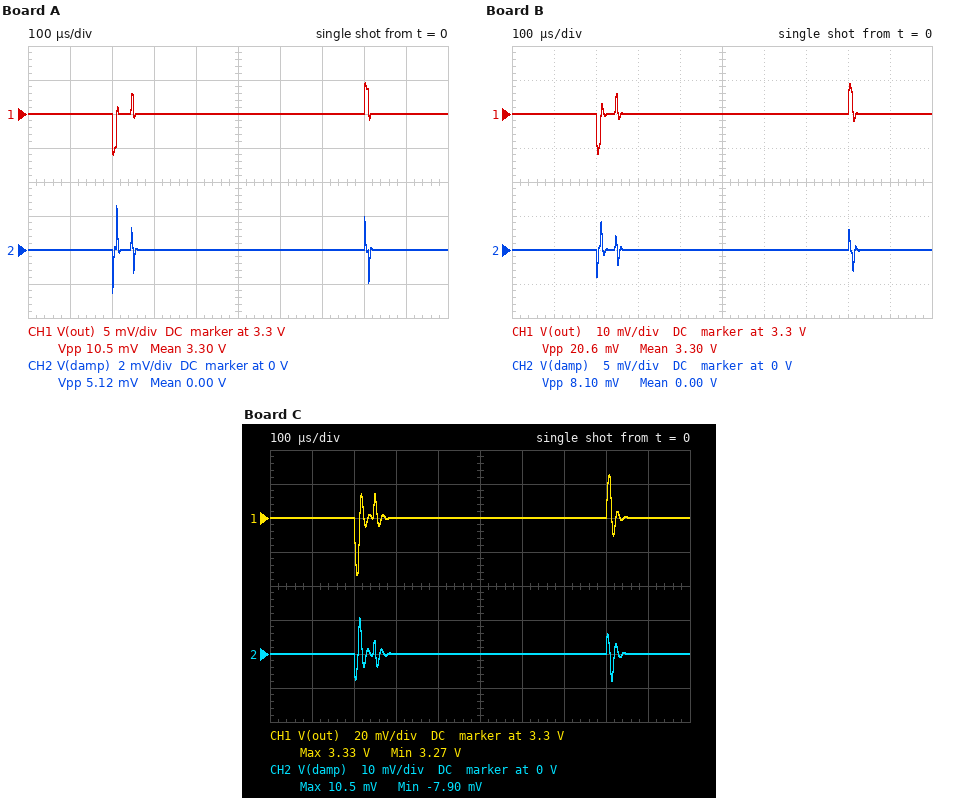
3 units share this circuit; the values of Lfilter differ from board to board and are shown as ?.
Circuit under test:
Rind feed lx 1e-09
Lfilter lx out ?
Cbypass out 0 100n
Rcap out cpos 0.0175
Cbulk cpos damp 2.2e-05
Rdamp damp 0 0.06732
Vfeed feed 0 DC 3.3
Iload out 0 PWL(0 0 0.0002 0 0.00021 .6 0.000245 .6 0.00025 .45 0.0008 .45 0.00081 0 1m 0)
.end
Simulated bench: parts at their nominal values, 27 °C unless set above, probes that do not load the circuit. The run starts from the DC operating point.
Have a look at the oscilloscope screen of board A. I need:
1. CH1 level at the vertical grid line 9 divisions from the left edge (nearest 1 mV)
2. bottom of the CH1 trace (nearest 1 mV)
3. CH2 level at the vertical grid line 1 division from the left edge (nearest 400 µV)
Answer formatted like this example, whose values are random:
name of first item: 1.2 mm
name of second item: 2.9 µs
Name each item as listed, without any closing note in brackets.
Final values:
CH1 level at the vertical grid line 9 divisions from the left edge: 3.300 V
bottom of the CH1 trace: 3.294 V
CH2 level at the vertical grid line 1 division from the left edge: 0 V
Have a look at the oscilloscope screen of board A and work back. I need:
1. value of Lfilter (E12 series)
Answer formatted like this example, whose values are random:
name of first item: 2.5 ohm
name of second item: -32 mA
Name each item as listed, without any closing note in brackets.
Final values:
value of Lfilter: 82 nH
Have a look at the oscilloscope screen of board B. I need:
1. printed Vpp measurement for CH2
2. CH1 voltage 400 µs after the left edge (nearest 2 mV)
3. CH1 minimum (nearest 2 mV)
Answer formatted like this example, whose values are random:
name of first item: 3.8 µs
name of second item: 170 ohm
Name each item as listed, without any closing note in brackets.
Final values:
printed Vpp measurement for CH2: 8.10 mV
CH1 voltage 400 µs after the left edge: 3.300 V
CH1 minimum: 3.288 V
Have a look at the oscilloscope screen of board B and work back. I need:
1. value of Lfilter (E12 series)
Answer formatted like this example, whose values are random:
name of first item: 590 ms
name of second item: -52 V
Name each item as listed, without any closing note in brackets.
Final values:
value of Lfilter: 150 nH
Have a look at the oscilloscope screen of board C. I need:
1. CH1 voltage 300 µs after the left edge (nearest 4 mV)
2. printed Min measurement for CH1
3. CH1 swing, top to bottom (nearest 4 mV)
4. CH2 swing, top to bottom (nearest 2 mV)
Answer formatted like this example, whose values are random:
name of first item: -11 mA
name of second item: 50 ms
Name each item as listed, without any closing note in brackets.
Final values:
CH1 voltage 300 µs after the left edge: 3.300 V
printed Min measurement for CH1: 3.27 V
CH1 swing, top to bottom: 60 mV
CH2 swing, top to bottom: 18 mV
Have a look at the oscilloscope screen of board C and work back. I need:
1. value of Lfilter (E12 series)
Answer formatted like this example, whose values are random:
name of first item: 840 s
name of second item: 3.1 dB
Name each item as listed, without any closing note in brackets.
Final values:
value of Lfilter: 390 nH
